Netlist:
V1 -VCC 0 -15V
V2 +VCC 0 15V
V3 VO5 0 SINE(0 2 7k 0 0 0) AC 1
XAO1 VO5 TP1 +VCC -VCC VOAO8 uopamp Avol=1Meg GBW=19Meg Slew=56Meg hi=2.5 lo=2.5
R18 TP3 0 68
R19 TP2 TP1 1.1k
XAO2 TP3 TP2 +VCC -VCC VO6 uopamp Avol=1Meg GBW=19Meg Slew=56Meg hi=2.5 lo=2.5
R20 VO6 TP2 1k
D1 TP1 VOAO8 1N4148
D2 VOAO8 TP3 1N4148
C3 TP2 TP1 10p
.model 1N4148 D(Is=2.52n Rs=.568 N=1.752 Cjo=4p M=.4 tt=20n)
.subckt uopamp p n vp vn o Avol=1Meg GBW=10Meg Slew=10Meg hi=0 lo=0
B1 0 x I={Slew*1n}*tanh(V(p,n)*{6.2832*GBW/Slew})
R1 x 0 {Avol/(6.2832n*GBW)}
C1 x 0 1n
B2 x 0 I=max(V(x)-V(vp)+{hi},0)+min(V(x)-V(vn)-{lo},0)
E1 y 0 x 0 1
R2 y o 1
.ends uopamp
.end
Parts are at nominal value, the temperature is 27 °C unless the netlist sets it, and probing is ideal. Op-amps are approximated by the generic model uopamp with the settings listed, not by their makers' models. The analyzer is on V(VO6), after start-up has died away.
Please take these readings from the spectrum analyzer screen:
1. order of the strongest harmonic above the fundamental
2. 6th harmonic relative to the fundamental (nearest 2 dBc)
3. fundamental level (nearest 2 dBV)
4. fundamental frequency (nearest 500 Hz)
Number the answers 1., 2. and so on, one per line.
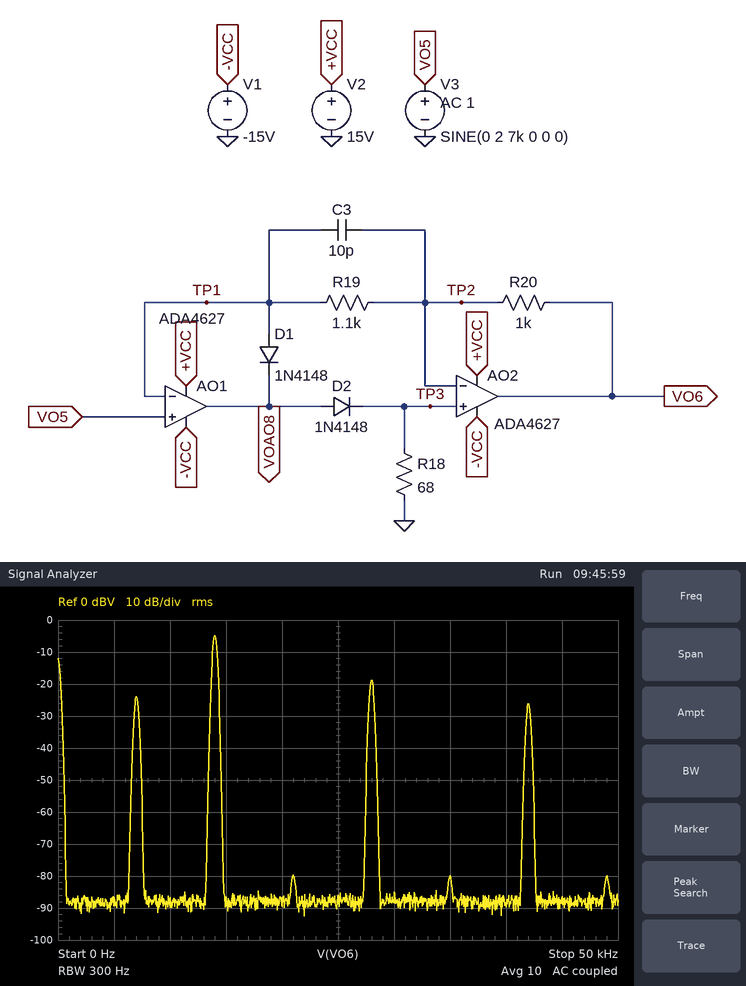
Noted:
1. 2
2. -2 dBc
3. -24 dBV
4. 7.0 kHz
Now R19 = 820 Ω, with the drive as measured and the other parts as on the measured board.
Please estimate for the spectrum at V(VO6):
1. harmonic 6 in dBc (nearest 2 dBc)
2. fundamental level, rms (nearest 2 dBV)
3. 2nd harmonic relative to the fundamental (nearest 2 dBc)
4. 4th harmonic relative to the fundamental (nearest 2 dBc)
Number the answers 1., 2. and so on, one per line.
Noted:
1. -8 dBc
2. -16 dBV
3. 12 dBc
4. -2 dBc
